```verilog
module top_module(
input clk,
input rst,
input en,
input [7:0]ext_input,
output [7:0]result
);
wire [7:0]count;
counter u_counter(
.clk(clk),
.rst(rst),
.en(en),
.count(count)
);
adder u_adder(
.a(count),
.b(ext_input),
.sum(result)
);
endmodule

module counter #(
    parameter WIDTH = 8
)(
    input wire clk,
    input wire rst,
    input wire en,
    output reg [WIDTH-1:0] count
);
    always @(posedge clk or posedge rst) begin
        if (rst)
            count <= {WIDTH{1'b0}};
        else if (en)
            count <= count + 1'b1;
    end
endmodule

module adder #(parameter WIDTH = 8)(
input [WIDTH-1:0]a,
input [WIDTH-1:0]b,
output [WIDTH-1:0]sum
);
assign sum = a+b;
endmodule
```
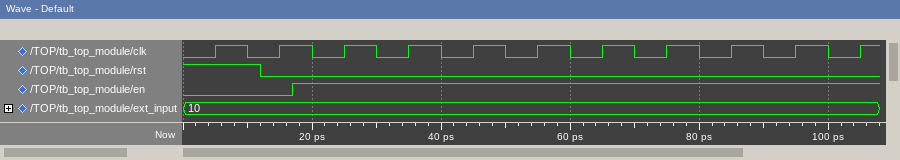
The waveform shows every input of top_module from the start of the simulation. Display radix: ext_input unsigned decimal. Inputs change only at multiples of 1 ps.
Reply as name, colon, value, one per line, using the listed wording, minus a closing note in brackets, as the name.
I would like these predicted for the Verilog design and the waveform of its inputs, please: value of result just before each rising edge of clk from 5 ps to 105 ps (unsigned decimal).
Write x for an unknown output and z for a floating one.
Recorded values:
value of result just before each rising edge of clk from 5 ps to 105 ps: 10, 10, 10, 11, 12, 13, 14, 15, 16, 17, 18
